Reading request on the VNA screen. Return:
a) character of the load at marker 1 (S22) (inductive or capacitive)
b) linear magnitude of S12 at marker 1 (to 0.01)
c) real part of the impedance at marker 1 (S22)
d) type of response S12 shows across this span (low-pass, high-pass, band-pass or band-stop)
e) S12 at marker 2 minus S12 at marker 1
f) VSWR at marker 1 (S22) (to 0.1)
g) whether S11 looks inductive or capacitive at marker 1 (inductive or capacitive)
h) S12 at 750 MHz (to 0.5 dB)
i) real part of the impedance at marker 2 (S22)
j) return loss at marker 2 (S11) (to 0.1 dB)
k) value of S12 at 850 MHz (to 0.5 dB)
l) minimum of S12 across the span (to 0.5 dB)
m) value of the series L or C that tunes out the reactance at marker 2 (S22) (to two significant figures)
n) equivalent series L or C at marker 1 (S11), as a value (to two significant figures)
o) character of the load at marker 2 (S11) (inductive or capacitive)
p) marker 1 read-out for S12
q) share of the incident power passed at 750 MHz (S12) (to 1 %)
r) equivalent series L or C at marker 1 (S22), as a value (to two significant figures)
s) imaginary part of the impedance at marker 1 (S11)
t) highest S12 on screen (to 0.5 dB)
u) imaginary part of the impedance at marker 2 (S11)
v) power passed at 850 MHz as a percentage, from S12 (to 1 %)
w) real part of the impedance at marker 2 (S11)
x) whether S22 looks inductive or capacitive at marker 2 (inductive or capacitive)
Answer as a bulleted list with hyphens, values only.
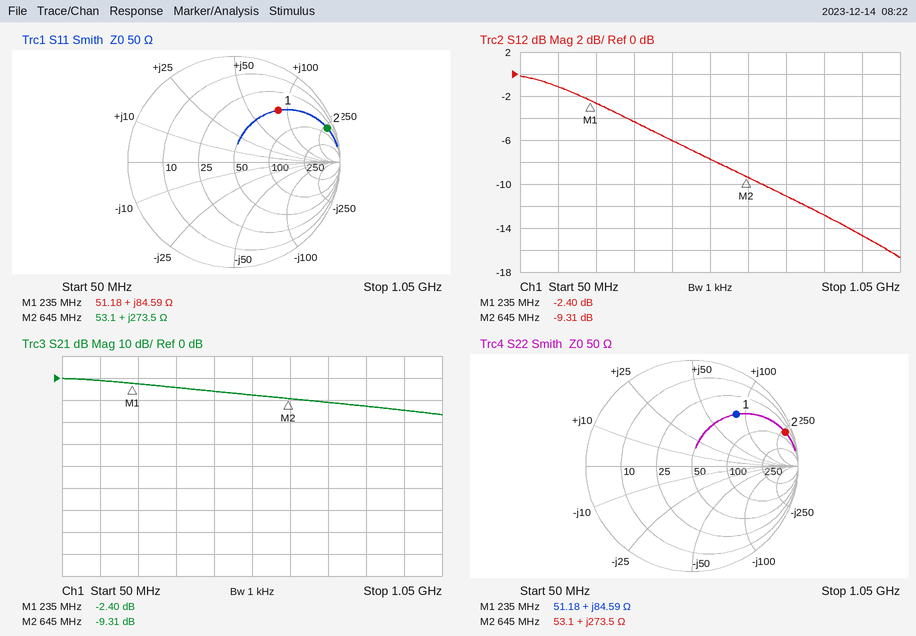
- inductive
- 0.76
- 51.18 Ω
- low-pass
- -6.91 dB
- 4.6
- inductive
- -11.0 dB
- 53.1 Ω
- 0.6 dB
- -13.0 dB
- -16.5 dB
- 900 fF
- 57 nH
- inductive
- -2.40 dB
- 8 %
- 57 nH
- +84.59 Ω
- 0.0 dB
- +273.5 Ω
- 5 %
- 53.1 Ω
- inductive
